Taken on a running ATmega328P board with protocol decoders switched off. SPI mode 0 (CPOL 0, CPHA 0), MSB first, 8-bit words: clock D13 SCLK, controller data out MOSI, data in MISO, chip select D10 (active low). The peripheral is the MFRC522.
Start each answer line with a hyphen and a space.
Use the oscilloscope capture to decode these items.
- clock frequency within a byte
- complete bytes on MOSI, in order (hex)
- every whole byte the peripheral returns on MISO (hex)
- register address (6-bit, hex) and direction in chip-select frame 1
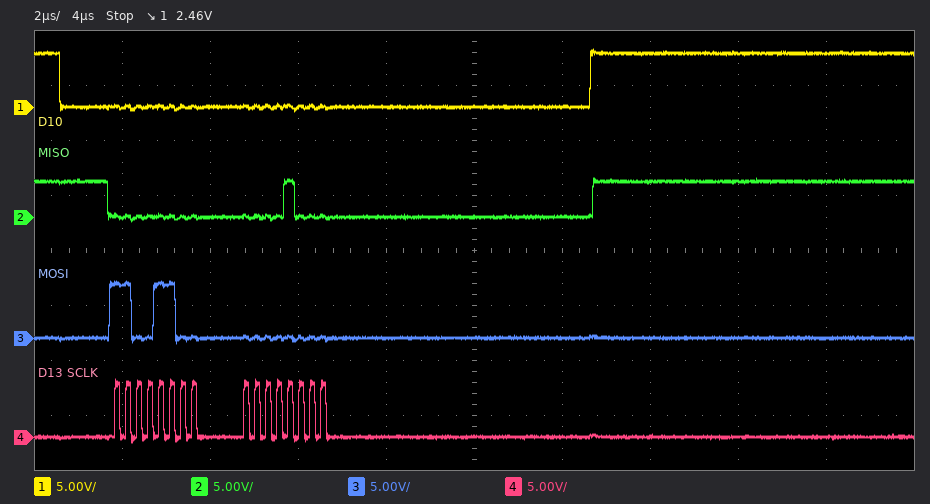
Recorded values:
- 4 MHz
- CC 00
- 00 08
- 0x26 read
